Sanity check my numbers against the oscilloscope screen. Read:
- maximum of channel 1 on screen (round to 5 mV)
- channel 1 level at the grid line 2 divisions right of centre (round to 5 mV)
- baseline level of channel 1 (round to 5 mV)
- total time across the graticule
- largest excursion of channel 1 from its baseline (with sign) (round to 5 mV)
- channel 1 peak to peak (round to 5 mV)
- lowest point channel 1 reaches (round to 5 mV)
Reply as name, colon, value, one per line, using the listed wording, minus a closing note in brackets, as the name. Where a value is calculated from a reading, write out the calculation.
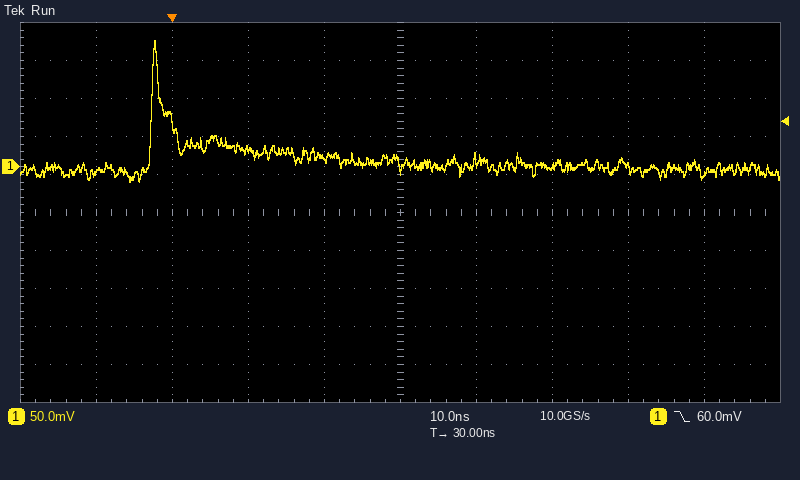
maximum of channel 1 on screen: 165 mV
channel 1 level at the grid line 2 divisions right of centre: 0 mV
baseline level of channel 1: 0 mV
total time across the graticule: 100 ns
largest excursion of channel 1 from its baseline (with sign): 165 mV − (0 mV) = +165 mV
channel 1 peak to peak: 165 mV − (-20 mV) = 185 mV
lowest point channel 1 reaches: -20 mV
